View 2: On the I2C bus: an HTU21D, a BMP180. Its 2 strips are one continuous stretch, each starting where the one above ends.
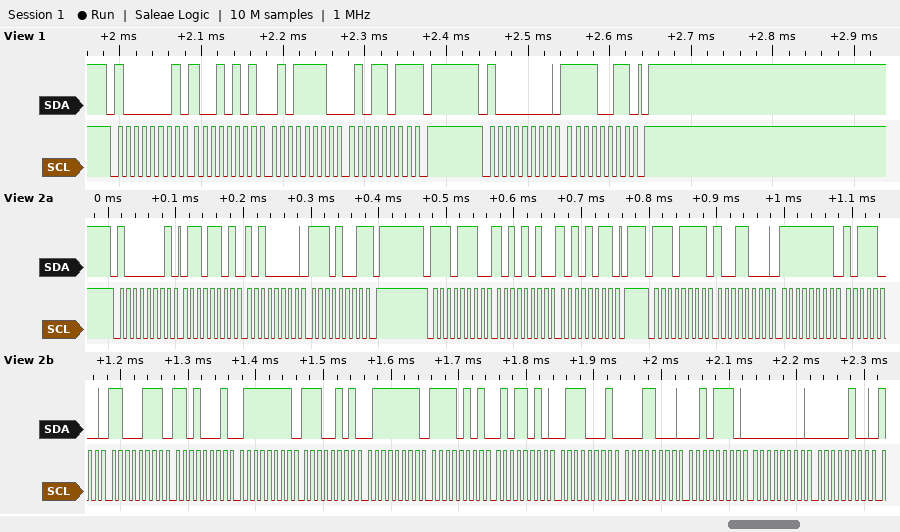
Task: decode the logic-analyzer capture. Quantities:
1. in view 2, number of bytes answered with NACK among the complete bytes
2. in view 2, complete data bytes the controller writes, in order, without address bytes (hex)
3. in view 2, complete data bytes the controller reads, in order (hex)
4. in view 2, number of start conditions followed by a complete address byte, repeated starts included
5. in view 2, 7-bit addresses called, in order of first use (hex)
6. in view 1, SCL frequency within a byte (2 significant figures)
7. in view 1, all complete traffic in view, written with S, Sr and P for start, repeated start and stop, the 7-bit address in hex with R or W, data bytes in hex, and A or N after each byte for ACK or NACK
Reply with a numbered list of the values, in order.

1. 1
2. AA AB
3. 6D A0 E9 98 FF B8 C7 D1 7F E5 7F F5 5A 71 18 2E 00 04
4. 3
5. 0x40 0x77
6. 100 kHz
7. S 40R A 95 A 5E A 5B N P S 40W A F3 A P
